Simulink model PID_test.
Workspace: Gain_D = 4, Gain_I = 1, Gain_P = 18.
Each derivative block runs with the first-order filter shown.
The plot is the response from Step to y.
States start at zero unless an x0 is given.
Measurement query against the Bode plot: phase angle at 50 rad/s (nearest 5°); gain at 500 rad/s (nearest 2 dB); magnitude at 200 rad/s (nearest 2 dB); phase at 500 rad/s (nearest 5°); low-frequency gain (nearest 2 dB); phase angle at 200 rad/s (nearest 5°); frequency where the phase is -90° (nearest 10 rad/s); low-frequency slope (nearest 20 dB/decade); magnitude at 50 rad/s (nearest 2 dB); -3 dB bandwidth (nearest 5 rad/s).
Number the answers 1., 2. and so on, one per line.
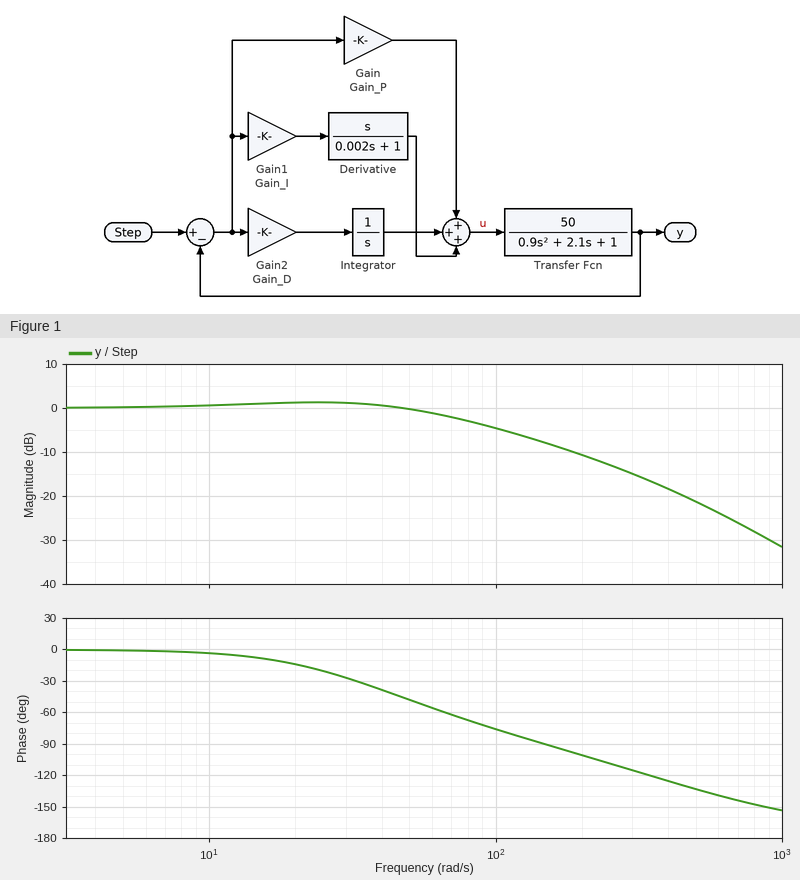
1. -50°
2. -22 dB
3. -10 dB
4. -135°
5. 0 dB
6. -100°
7. 150 rad/s
8. 0 dB/decade
9. 0 dB
10. 80 rad/s
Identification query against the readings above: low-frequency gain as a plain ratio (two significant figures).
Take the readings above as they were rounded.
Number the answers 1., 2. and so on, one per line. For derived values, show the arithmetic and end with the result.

1. 10^(0 / 20) = 1.0
